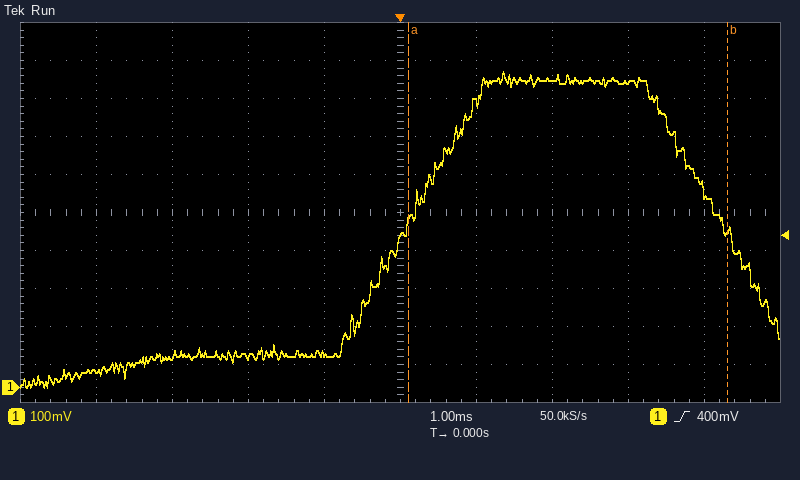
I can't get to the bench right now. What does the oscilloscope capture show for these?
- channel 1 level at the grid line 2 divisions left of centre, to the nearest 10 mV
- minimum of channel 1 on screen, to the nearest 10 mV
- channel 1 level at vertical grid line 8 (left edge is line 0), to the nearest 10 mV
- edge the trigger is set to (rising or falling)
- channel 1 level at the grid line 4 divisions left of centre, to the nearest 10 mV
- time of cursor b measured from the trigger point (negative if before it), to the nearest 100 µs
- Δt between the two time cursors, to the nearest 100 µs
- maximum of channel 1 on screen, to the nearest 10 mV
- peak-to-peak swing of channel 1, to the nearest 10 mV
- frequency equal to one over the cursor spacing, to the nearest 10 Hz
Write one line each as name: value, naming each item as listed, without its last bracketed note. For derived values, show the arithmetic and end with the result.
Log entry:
channel 1 level at the grid line 2 divisions left of centre, to the nearest 10 mV: 80 mV
minimum of channel 1 on screen, to the nearest 10 mV: 0 mV
channel 1 level at vertical grid line 8 (left edge is line 0), to the nearest 10 mV: 800 mV
edge the trigger is set to: rising
channel 1 level at the grid line 4 divisions left of centre, to the nearest 10 mV: 40 mV
time of cursor b measured from the trigger point (negative if before it), to the nearest 100 µs: +4.3 ms
Δt between the two time cursors, to the nearest 100 µs: 4.2 ms
maximum of channel 1 on screen, to the nearest 10 mV: 830 mV
peak-to-peak swing of channel 1, to the nearest 10 mV: 830 mV − (0 mV) = 830 mV
frequency equal to one over the cursor spacing, to the nearest 10 Hz: 1 / 4.2 ms ≈ 240 Hz
